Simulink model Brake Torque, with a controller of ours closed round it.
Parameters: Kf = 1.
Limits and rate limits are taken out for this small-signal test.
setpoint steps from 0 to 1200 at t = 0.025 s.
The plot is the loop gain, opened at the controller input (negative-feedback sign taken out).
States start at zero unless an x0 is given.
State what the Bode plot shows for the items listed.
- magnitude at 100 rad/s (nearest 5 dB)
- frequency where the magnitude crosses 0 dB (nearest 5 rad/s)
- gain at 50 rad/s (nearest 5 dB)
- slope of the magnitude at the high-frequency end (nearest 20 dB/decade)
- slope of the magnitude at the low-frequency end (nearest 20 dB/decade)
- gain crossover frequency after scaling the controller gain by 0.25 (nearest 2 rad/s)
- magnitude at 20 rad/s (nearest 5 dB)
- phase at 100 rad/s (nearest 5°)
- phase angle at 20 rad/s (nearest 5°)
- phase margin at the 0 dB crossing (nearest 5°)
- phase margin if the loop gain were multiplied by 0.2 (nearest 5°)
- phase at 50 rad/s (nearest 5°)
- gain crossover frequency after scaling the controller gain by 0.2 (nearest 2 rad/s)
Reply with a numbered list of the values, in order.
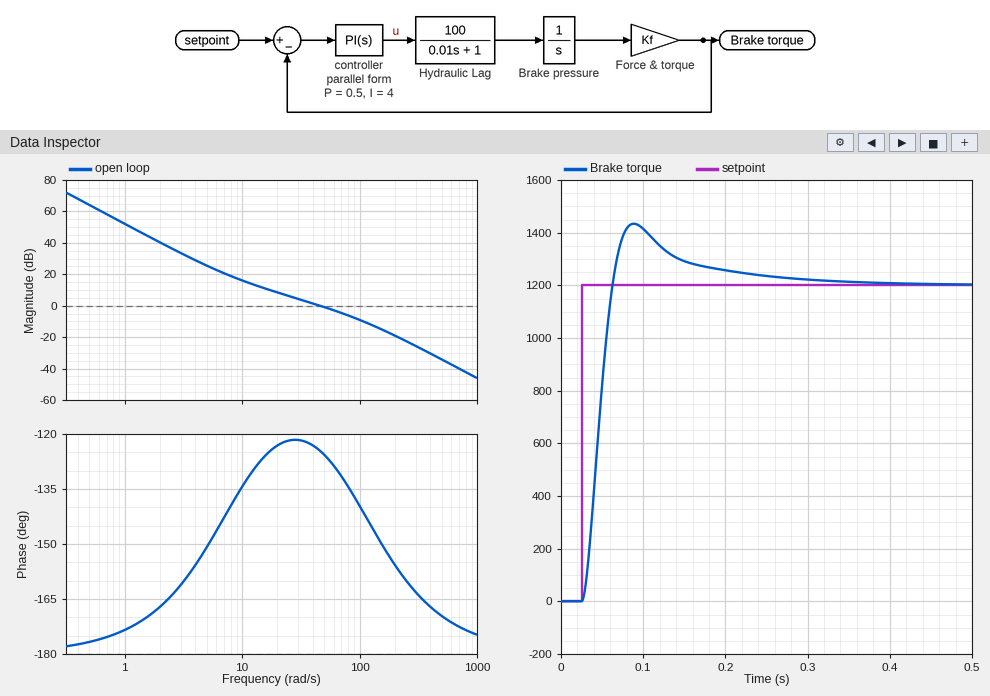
1. -10 dB
2. 45 rad/s
3. 0 dB
4. -40 dB/decade
5. -40 dB/decade
6. 14 rad/s
7. 10 dB
8. -140°
9. -125°
10. 55°
11. 50°
12. -125°
13. 12 rad/s
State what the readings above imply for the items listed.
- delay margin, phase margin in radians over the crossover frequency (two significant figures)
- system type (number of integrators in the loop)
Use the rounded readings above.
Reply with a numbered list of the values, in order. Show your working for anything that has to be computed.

1. 55 × π / 180 / 45 = 0.021 s
2. 2
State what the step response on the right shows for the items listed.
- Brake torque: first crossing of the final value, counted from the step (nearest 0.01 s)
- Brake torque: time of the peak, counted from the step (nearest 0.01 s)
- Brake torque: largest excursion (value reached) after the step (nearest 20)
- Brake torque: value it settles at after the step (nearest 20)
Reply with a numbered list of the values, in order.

1. 0.04 s
2. 0.06 s
3. 1440
4. 1200
